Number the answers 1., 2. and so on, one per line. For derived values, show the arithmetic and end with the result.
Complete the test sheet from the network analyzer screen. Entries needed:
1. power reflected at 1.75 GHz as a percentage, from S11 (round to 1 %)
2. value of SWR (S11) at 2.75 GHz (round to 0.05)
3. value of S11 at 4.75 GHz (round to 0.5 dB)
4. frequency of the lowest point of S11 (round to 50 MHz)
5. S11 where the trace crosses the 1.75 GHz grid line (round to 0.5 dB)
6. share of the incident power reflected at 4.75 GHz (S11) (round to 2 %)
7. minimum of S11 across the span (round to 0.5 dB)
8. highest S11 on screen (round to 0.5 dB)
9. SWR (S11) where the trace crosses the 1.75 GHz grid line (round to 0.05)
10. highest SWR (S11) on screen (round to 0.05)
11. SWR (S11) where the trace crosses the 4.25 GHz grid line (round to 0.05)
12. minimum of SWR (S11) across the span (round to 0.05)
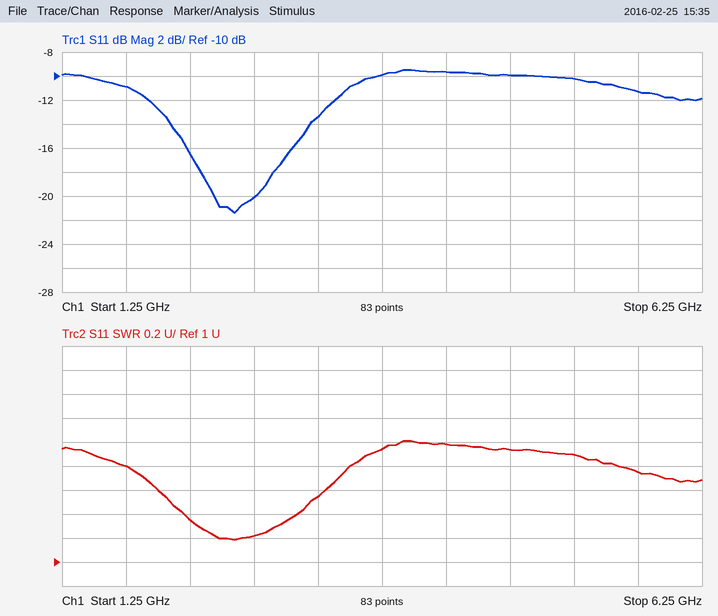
1. 10^(-11/10) ≈ 8 %
2. 1.20
3. -10.0 dB
4. 2.60 GHz
5. -11.0 dB
6. 10^(-10/10) ≈ 10 %
7. -21.5 dB
8. -9.5 dB
9. 1.80
10. 2.00
11. 2.00
12. 1.20
